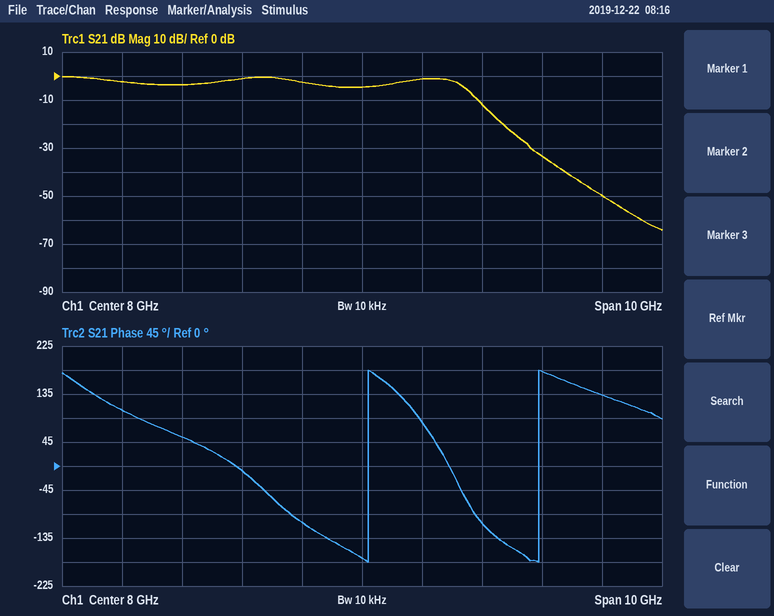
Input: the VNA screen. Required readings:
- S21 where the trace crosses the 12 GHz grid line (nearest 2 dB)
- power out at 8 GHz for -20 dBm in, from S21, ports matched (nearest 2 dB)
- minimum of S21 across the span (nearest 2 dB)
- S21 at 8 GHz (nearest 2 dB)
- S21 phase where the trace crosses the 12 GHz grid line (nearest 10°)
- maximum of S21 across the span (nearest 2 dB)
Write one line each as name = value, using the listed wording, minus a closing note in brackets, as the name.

S21 where the trace crosses the 12 GHz grid line = -50 dB
power out at 8 GHz for -20 dBm in, from S21, ports matched = -24 dBm
minimum of S21 across the span = -64 dB
S21 at 8 GHz = -4 dB
S21 phase where the trace crosses the 12 GHz grid line = 130°
maximum of S21 across the span = 0 dB
